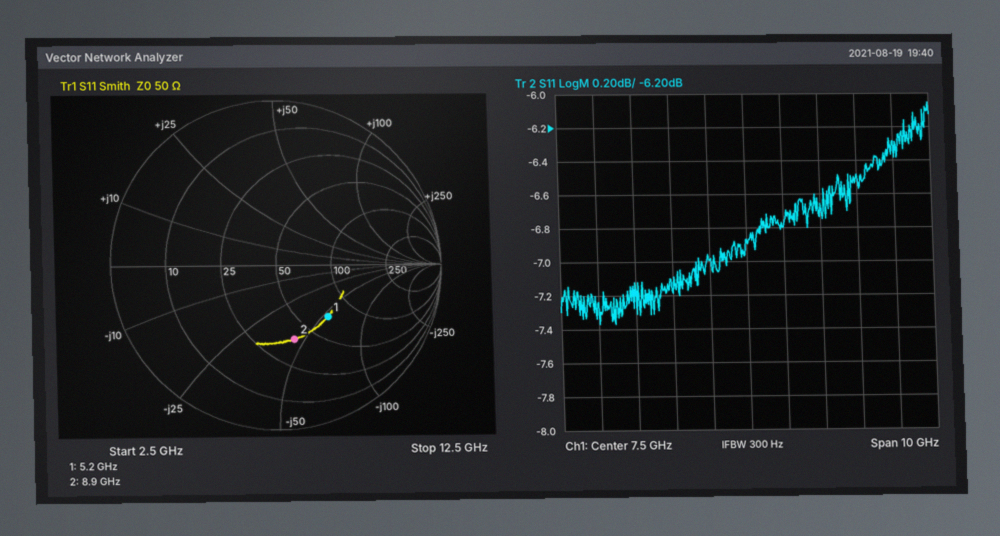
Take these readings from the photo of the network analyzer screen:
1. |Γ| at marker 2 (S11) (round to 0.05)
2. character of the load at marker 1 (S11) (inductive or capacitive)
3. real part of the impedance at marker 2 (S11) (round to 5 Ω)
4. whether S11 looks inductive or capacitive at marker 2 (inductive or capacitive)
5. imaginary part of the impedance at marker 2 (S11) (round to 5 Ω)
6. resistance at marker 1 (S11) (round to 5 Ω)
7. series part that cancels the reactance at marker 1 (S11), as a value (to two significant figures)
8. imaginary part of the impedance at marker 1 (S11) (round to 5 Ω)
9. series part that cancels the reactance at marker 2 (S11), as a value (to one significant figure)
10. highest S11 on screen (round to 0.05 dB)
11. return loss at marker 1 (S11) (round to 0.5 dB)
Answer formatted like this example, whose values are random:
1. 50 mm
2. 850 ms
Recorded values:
1. 0.45
2. capacitive
3. 40 Ω
4. capacitive
5. -45 Ω
6. 70 Ω
7. 1.7 nH
8. -55 Ω
9. 800 pH
10. -6.05 dB
11. 7.0 dB
